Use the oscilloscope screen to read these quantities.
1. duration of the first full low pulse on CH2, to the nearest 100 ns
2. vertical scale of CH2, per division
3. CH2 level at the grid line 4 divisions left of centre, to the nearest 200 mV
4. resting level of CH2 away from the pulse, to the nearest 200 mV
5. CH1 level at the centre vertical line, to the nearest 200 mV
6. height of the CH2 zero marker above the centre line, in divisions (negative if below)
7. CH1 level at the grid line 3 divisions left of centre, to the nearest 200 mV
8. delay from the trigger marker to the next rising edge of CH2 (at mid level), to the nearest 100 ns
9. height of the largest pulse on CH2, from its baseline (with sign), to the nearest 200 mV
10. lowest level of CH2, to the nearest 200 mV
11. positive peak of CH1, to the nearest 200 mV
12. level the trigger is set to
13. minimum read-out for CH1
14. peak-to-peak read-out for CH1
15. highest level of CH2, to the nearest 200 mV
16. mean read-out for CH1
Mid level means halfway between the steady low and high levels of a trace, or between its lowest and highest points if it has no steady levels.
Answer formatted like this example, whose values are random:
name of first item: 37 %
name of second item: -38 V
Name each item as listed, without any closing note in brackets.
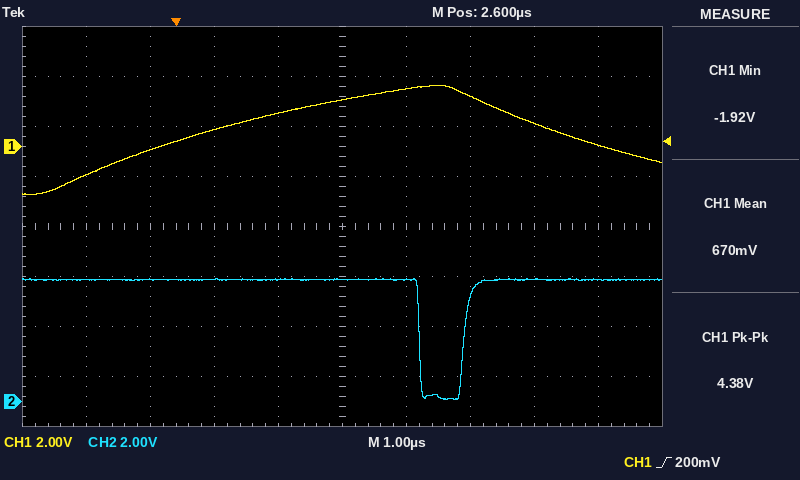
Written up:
duration of the first full low pulse on CH2, to the nearest 100 ns: 700 ns
vertical scale of CH2, per division: 2 V
CH2 level at the grid line 4 divisions left of centre, to the nearest 200 mV: 4.8 V
resting level of CH2 away from the pulse, to the nearest 200 mV: 4.8 V
CH1 level at the centre vertical line, to the nearest 200 mV: 1.8 V
height of the CH2 zero marker above the centre line, in divisions: -3.5 div
CH1 level at the grid line 3 divisions left of centre, to the nearest 200 mV: -200 mV
delay from the trigger marker to the next rising edge of CH2 (at mid level), to the nearest 100 ns: 4.5 µs
height of the largest pulse on CH2, from its baseline (with sign), to the nearest 200 mV: -4.8 V
lowest level of CH2, to the nearest 200 mV: 0.0 V
positive peak of CH1, to the nearest 200 mV: 2.4 V
level the trigger is set to: 200 mV
minimum read-out for CH1: -1.92 V
peak-to-peak read-out for CH1: 4.38 V
highest level of CH2, to the nearest 200 mV: 5.0 V
mean read-out for CH1: 670 mV
